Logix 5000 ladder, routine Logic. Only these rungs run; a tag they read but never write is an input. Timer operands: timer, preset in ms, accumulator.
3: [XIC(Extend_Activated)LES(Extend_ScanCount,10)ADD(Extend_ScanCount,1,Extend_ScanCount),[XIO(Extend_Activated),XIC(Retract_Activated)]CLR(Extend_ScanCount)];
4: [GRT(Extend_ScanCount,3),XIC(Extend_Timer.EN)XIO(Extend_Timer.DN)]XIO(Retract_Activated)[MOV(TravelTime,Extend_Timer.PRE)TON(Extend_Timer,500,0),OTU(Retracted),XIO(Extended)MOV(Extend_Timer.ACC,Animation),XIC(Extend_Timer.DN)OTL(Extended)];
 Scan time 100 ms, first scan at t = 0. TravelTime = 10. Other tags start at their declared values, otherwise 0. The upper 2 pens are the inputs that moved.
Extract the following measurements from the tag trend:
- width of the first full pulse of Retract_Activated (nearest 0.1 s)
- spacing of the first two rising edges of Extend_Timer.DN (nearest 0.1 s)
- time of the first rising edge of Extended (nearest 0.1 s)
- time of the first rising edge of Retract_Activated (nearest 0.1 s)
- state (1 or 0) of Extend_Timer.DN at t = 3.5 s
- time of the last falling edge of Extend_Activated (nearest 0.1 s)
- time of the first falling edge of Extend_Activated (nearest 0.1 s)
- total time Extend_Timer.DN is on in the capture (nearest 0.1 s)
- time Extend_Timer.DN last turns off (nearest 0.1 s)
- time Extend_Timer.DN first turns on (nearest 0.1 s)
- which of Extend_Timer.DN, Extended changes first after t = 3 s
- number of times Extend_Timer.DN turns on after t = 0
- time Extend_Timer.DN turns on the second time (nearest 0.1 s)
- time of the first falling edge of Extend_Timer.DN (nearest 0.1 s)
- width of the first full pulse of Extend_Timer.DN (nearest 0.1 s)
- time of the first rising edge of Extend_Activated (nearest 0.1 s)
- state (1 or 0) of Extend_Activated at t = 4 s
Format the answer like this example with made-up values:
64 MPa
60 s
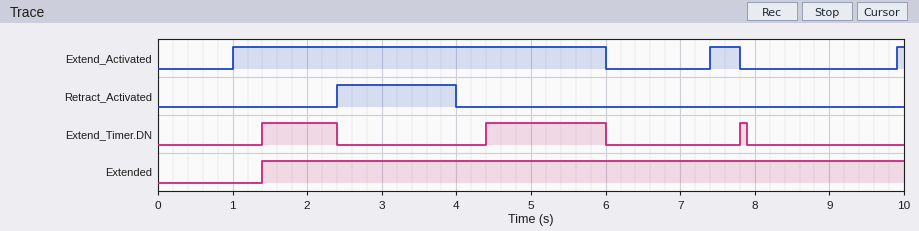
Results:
1.6 s
3.0 s
1.4 s
2.4 s
0
7.8 s
6.0 s
2.7 s
7.9 s
1.4 s
Extend_Timer.DN
3
4.4 s
2.4 s
1.0 s
1.0 s
1
